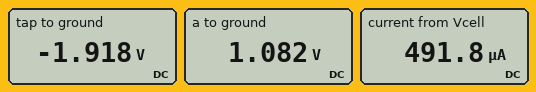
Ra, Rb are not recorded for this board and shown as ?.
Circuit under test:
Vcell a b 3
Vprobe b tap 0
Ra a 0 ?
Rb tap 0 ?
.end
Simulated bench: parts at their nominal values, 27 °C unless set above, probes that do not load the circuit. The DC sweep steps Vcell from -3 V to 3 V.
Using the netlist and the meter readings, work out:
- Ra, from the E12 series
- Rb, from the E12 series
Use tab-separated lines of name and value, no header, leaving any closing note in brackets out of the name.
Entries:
Ra, from the E12 series	2.2 kΩ
Rb, from the E12 series	3.9 kΩ
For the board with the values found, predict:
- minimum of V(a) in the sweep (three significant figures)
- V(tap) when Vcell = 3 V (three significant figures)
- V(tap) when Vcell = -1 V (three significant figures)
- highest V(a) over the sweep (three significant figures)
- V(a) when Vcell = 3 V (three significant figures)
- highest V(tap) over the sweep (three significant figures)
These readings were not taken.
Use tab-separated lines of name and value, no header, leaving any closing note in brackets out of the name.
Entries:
minimum of V(a) in the sweep	-1.08 V
V(tap) when Vcell = 3 V	-1.92 V
V(tap) when Vcell = -1 V	639 mV
highest V(a) over the sweep	1.08 V
V(a) when Vcell = 3 V	1.08 V
highest V(tap) over the sweep	1.92 V
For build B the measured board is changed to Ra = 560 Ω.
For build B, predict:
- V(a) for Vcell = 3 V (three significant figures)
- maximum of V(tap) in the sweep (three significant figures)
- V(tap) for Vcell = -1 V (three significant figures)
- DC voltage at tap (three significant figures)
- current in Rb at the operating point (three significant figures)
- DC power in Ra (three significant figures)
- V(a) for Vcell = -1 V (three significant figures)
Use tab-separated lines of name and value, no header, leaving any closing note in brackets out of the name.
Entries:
V(a) for Vcell = 3 V	377 mV
maximum of V(tap) in the sweep	2.62 V
V(tap) for Vcell = -1 V	874 mV
DC voltage at tap	-2.62 V
current in Rb at the operating point	673 µA
DC power in Ra	253 µW
V(a) for Vcell = -1 V	-126 mV
